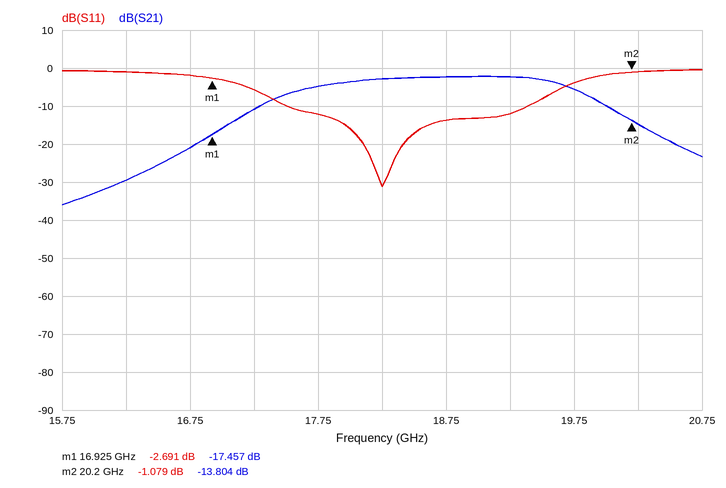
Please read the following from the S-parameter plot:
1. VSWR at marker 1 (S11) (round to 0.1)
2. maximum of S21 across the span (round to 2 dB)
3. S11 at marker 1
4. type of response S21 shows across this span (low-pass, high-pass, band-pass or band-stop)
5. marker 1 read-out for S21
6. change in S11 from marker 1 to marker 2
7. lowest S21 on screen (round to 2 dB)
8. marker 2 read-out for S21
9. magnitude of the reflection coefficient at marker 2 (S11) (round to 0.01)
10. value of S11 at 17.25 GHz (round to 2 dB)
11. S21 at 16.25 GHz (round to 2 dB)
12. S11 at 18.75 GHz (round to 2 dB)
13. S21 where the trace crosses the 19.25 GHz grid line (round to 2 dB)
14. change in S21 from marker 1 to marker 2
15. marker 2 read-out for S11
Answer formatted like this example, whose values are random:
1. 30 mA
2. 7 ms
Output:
1. 6.5
2. -2 dB
3. -2.691 dB
4. band-pass
5. -17.457 dB
6. 1.612 dB
7. -36 dB
8. -13.804 dB
9. 0.88
10. -6 dB
11. -30 dB
12. -14 dB
13. -2 dB
14. 3.653 dB
15. -1.079 dB
